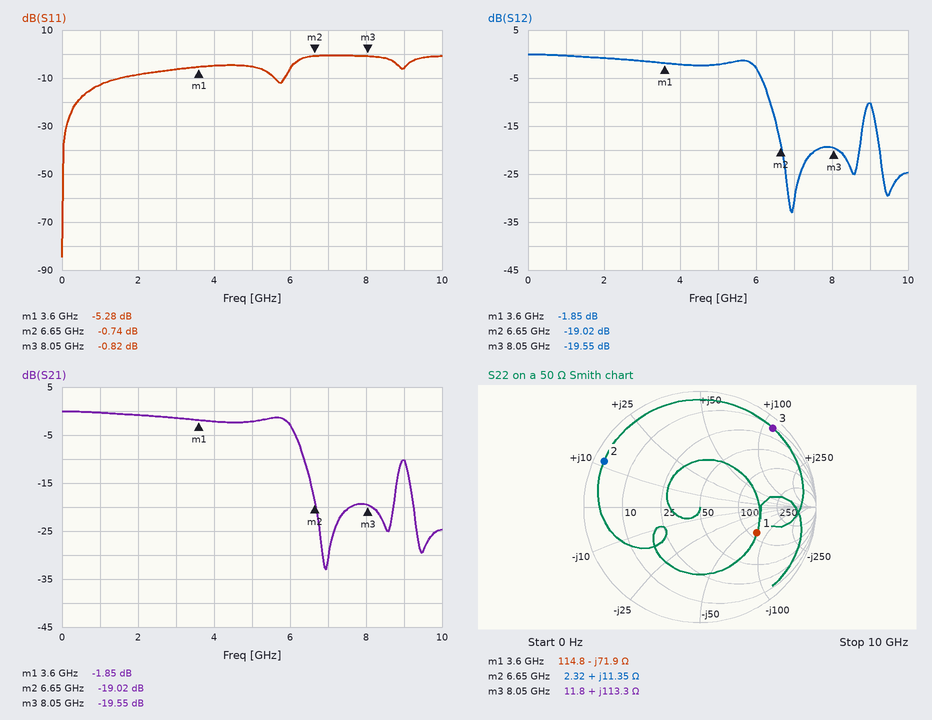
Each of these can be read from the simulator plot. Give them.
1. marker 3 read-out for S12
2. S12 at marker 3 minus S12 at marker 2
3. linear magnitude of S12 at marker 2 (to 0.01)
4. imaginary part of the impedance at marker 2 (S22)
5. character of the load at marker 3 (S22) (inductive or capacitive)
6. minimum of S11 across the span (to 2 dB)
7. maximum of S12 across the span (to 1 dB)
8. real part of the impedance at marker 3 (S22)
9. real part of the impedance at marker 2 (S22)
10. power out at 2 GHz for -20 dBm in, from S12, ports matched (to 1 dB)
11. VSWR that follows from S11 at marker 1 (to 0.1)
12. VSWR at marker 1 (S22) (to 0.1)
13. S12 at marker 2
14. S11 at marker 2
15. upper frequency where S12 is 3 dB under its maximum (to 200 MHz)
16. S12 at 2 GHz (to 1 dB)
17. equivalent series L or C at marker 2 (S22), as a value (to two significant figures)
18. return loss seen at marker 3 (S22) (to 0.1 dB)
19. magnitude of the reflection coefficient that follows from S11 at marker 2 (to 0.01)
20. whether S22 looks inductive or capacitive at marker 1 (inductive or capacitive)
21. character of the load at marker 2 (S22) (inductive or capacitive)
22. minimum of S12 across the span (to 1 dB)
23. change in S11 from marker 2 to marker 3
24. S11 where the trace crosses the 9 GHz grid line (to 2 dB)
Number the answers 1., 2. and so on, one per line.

1. -19.55 dB
2. -0.53 dB
3. 0.11
4. +11.35 Ω
5. inductive
6. -84 dB
7. 0 dB
8. 11.8 Ω
9. 2.32 Ω
10. -21 dBm
11. 3.4
12. 3.3
13. -19.02 dB
14. -0.74 dB
15. 6.0 GHz
16. -1 dB
17. 270 pH
18. 0.7 dB
19. 0.92
20. capacitive
21. inductive
22. -33 dB
23. -0.08 dB
24. -6 dB
